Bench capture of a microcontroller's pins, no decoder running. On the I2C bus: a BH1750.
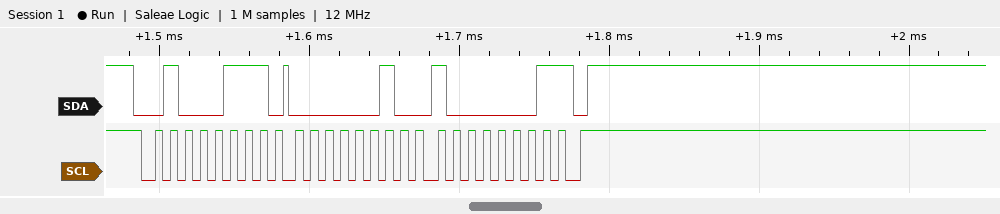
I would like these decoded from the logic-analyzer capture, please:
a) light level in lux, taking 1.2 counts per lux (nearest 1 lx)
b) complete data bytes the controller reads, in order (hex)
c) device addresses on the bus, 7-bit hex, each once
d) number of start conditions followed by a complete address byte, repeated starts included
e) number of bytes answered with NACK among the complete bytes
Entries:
534 lx
02 81
0x23
1
1
